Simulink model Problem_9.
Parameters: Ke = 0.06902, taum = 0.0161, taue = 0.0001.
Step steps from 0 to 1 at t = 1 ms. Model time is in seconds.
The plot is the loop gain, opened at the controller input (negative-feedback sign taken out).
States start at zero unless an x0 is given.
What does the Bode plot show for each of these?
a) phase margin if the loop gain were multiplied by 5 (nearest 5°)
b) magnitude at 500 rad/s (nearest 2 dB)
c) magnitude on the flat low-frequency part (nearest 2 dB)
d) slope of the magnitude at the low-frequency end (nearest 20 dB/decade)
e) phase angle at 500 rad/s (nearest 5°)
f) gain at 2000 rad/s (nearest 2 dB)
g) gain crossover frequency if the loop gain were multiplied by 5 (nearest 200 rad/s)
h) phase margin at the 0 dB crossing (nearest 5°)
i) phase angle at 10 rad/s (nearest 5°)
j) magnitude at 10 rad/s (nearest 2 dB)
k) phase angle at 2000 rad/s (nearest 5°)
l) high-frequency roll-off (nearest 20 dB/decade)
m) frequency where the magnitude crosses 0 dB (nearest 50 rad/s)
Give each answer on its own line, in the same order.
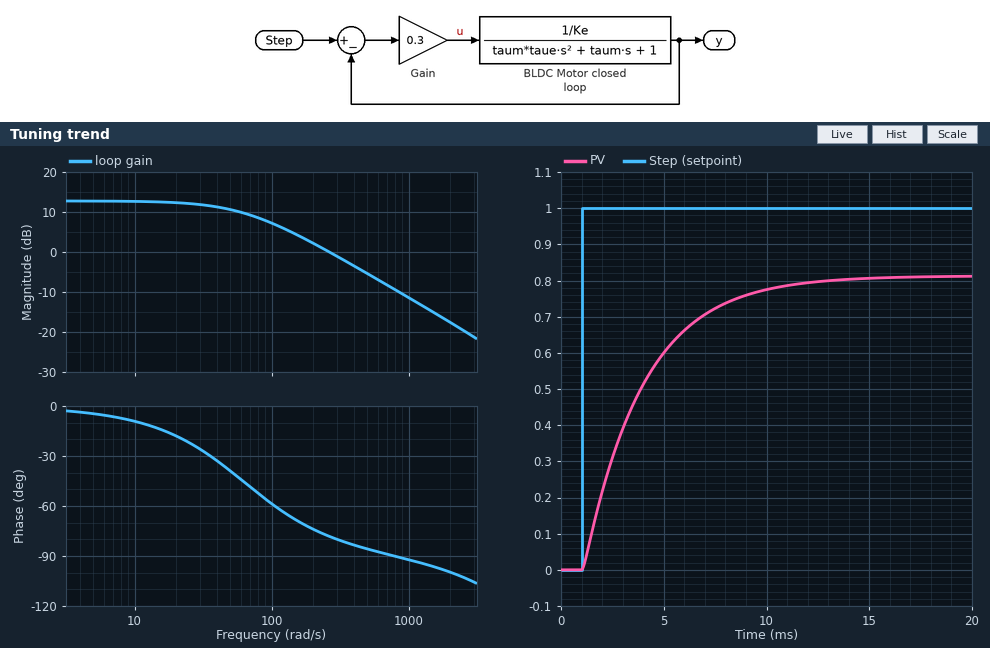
85°
-6 dB
12 dB
0 dB/decade
-85°
-18 dB
1400 rad/s
100°
-10°
12 dB
-100°
-20 dB/decade
250 rad/s
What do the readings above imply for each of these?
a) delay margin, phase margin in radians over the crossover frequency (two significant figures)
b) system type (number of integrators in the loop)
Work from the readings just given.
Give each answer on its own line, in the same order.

0.0070 s
0
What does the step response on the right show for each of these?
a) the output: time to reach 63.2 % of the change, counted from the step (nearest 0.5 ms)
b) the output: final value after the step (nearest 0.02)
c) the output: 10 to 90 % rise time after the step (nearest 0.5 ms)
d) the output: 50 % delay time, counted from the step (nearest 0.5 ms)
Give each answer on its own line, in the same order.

3.0 ms
0.82
6.5 ms
2.0 ms
